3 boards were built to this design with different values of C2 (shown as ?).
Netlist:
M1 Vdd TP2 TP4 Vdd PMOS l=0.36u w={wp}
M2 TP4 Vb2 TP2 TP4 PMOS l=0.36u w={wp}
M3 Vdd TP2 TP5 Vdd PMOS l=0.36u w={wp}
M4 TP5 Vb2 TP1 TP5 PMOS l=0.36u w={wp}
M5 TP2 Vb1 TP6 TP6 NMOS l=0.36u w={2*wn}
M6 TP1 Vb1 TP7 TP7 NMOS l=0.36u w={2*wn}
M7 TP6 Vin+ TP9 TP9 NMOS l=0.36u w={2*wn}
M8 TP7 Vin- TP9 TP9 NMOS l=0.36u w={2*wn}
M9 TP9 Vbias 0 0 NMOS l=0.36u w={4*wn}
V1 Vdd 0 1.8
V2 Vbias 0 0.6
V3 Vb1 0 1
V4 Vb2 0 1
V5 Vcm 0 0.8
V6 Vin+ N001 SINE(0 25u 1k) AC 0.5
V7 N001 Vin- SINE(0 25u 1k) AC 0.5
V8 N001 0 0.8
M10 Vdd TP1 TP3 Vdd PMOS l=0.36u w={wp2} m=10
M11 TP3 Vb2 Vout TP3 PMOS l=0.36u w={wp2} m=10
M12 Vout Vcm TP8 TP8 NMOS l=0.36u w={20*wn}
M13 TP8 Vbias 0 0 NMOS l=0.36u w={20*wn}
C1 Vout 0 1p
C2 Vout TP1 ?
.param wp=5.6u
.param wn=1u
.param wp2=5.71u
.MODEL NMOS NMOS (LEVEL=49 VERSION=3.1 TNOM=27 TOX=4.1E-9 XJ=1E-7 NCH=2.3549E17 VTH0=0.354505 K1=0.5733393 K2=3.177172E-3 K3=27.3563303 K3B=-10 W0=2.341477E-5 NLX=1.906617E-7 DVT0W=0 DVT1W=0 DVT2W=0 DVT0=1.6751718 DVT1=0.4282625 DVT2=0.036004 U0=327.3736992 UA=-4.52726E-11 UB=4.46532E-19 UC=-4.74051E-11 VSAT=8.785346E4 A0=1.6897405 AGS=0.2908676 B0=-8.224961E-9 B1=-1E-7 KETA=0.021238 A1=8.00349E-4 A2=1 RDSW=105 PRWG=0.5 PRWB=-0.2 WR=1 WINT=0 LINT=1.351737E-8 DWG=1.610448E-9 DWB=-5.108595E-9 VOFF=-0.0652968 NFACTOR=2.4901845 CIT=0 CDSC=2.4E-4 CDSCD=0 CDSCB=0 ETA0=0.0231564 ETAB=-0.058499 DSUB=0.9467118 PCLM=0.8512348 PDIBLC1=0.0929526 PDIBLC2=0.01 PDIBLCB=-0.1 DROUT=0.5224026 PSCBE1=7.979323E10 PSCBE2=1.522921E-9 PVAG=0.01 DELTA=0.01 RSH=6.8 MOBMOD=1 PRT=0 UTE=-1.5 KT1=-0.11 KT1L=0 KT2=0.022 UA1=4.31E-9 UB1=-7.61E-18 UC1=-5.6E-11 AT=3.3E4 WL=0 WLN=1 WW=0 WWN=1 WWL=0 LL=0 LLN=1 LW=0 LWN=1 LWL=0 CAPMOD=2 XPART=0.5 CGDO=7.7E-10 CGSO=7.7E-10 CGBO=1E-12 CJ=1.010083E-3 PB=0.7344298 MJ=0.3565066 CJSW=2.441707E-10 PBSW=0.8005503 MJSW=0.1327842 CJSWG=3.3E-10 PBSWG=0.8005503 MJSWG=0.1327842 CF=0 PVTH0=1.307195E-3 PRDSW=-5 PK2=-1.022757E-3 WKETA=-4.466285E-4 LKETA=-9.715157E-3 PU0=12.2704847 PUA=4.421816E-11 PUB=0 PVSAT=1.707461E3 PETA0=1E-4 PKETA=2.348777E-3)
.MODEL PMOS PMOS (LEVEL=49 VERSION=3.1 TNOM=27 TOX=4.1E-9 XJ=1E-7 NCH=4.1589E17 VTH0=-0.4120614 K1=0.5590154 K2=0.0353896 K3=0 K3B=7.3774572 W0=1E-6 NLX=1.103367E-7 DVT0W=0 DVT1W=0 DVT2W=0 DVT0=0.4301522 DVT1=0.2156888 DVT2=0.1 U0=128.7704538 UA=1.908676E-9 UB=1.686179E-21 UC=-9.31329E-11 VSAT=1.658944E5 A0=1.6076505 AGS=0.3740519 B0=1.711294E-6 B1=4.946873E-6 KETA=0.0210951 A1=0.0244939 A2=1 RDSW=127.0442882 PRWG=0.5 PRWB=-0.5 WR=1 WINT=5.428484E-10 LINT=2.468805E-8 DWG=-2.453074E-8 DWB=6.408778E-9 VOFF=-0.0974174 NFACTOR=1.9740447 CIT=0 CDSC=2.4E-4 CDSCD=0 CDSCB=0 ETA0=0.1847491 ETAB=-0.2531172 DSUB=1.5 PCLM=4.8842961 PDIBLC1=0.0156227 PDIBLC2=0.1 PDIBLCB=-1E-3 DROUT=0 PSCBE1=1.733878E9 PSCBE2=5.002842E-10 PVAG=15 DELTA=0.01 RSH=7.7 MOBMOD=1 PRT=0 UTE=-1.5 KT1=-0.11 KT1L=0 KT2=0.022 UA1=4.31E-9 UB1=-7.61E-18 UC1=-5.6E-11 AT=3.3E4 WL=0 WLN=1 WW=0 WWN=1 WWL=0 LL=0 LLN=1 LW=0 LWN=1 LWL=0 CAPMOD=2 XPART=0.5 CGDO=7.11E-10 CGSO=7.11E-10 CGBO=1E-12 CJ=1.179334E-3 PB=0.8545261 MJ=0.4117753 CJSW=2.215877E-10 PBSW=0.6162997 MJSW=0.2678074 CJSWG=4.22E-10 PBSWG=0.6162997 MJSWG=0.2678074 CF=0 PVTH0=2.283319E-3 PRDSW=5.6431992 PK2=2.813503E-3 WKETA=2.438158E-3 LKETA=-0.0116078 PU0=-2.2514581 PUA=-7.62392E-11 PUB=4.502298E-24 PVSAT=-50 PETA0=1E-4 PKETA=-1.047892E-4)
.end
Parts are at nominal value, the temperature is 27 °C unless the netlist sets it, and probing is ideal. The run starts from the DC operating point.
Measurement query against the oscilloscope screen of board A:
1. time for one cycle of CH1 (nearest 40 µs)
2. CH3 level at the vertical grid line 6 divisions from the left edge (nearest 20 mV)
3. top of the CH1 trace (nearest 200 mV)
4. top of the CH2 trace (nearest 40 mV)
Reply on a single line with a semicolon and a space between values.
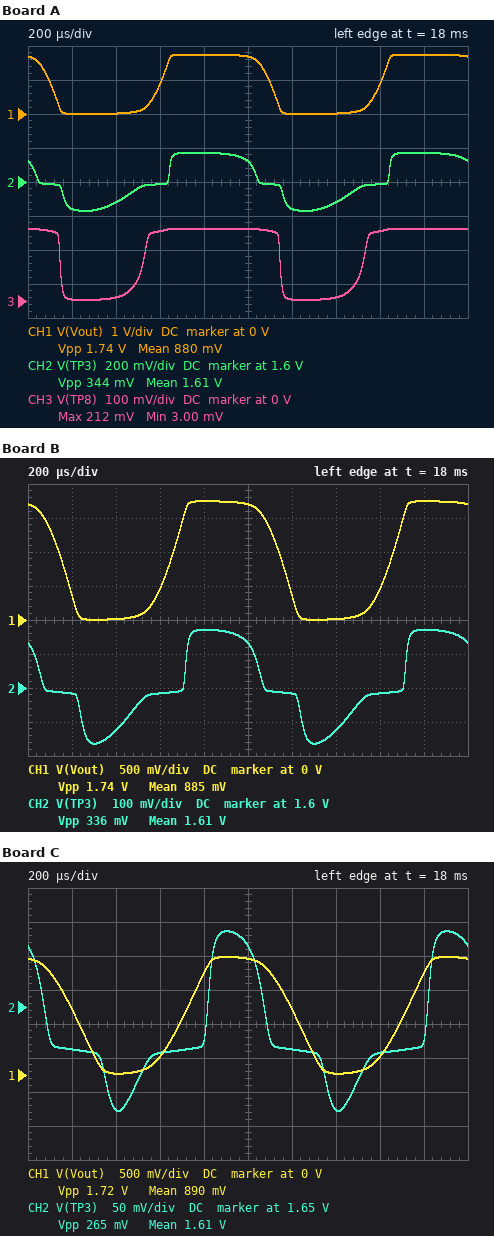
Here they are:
1.00 ms; 0 V; 1.8 V; 1.76 V
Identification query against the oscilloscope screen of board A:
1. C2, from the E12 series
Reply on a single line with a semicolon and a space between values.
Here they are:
270 fF
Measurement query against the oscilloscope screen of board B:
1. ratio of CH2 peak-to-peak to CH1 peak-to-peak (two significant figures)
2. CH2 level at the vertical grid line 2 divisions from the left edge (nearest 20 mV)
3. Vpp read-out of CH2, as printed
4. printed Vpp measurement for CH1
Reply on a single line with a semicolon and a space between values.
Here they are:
0.19; 1.48 V; 336 mV; 1.74 V
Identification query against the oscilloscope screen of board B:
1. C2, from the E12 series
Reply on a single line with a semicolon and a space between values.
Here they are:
560 fF
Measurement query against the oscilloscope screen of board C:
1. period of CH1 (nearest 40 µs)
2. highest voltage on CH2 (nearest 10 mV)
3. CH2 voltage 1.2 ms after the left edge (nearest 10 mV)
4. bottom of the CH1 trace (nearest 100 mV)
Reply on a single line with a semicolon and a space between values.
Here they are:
1.00 ms; 1.76 V; 1.59 V; 0 V
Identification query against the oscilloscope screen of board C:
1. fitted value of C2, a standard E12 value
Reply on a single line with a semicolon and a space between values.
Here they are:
1 pF
